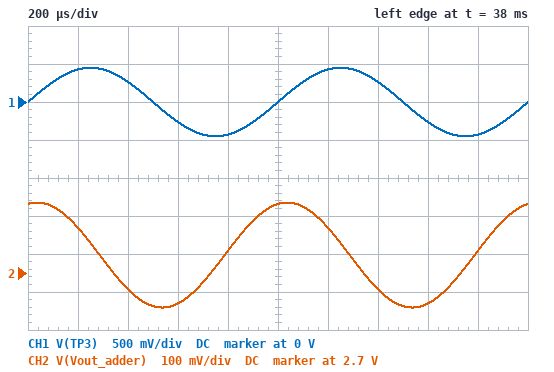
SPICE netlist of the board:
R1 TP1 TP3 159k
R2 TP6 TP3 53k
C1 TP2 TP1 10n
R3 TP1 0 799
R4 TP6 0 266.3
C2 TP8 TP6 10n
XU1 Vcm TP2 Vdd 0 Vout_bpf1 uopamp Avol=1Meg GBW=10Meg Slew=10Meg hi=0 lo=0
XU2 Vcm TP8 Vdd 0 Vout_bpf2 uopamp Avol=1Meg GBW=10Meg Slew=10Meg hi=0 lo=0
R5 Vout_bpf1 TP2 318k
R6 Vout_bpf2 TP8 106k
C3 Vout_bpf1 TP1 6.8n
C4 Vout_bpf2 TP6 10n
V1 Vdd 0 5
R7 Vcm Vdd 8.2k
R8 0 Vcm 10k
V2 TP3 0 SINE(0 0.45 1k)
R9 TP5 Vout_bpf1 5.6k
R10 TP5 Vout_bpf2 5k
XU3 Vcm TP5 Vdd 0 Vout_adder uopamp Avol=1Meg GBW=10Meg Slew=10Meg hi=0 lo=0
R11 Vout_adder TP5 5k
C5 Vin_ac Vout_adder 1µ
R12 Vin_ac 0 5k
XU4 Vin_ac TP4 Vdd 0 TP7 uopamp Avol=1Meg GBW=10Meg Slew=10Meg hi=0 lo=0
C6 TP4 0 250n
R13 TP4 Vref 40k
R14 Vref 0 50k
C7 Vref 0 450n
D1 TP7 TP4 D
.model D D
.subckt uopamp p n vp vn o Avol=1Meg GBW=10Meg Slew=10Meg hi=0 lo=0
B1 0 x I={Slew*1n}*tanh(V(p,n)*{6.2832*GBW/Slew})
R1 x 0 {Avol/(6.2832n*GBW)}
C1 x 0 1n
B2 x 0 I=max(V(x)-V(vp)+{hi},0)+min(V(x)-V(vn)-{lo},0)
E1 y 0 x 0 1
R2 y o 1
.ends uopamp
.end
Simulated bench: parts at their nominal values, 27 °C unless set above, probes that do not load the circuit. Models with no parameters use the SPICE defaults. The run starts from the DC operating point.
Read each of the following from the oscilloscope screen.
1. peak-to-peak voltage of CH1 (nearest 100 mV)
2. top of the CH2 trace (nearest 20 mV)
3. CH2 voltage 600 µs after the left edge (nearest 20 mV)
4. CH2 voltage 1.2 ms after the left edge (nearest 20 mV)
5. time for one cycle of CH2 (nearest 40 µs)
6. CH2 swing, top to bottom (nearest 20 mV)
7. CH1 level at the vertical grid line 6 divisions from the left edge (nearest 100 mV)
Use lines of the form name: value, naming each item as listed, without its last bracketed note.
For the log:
peak-to-peak voltage of CH1: 900 mV
top of the CH2 trace: 2.88 V
CH2 voltage 600 µs after the left edge: 2.62 V
CH2 voltage 1.2 ms after the left edge: 2.82 V
time for one cycle of CH2: 1.00 ms
CH2 swing, top to bottom: 280 mV
CH1 level at the vertical grid line 6 divisions from the left edge: 400 mV
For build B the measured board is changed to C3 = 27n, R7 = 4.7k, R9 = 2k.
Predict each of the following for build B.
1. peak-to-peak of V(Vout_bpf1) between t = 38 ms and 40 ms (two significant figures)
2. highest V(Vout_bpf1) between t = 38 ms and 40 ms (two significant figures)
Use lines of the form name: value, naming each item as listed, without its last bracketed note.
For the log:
peak-to-peak of V(Vout_bpf1) between t = 38 ms and 40 ms: 53 mV
highest V(Vout_bpf1) between t = 38 ms and 40 ms: 3.4 V
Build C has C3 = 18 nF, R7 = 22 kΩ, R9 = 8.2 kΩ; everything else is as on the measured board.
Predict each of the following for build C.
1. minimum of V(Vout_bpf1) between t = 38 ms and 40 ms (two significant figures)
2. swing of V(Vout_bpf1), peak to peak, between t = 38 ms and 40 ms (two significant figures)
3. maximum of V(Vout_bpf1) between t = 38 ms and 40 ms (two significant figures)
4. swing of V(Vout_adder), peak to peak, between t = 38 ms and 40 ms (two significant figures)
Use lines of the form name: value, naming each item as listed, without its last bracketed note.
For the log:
minimum of V(Vout_bpf1) between t = 38 ms and 40 ms: 1.5 V
swing of V(Vout_bpf1), peak to peak, between t = 38 ms and 40 ms: 110 mV
maximum of V(Vout_bpf1) between t = 38 ms and 40 ms: 1.6 V
swing of V(Vout_adder), peak to peak, between t = 38 ms and 40 ms: 35 mV
